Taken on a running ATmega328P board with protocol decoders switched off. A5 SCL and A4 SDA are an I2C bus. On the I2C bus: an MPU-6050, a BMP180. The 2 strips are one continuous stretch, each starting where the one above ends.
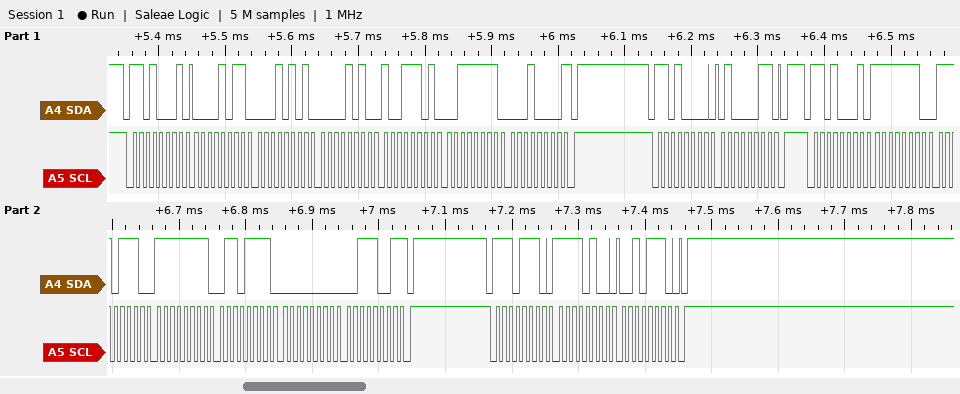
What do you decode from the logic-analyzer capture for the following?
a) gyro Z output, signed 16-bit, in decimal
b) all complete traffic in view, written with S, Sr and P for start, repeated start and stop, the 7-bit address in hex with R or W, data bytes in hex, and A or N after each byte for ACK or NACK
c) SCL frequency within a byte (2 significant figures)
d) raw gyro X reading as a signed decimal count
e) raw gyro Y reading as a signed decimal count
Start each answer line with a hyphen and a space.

- 57
- S 68R A 0B A 15 A 0A A 9D A 3F A 10 N P S 68W A 43 A P S 68R A FE A EE A FF A 6F A 00 A 39 N P S 77W A F4 A 2E A P
- 100 kHz
- -274
- -145
